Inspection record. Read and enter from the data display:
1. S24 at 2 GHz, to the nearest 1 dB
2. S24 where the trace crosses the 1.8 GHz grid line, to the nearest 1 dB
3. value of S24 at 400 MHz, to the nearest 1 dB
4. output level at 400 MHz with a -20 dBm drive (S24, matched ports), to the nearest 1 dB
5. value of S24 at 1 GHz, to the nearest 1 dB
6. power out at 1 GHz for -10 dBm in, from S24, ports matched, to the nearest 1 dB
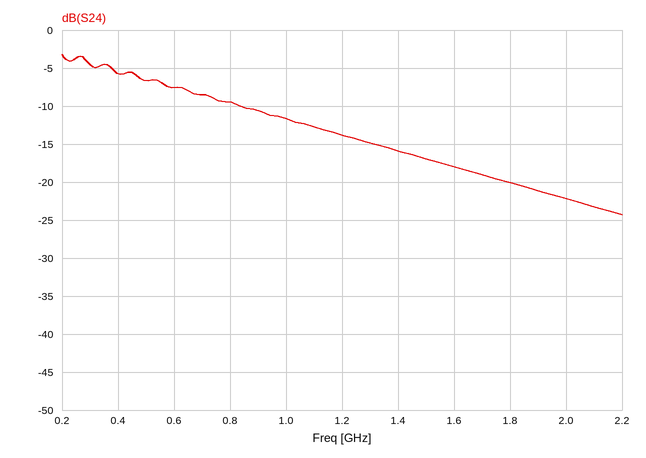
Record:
-22 dB
-20 dB
-6 dB
-26 dBm
-12 dB
-22 dBm
